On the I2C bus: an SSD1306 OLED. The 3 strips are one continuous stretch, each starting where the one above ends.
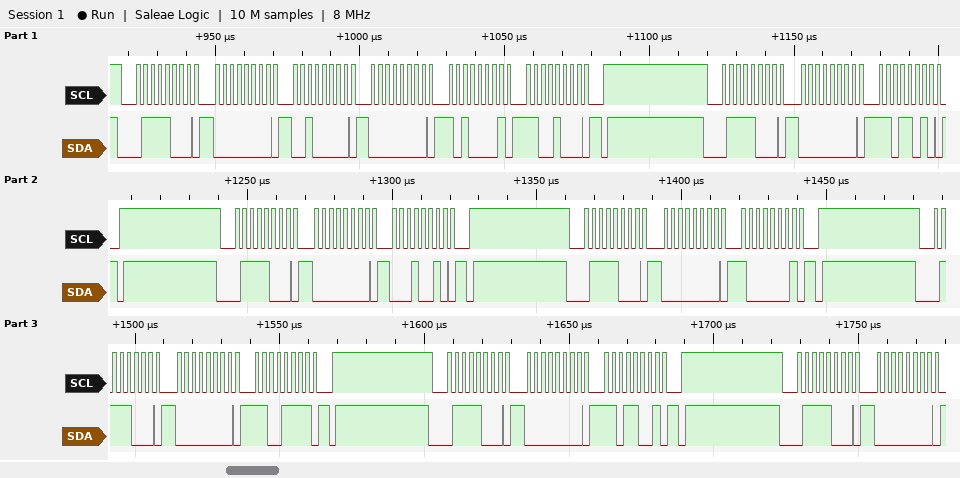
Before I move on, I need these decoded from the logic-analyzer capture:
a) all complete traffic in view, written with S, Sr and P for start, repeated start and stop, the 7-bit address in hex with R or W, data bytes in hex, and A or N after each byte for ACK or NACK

S 3CW A 00 A 20 A 00 A A1 A C8 A P S 3CW A 00 A DA A P S 3CW A 00 A 12 A P S 3CW A 00 A 81 A P S 3CW A 00 A CF A P S 3CW A 00 A D9 A P S 3CW A 00 A
